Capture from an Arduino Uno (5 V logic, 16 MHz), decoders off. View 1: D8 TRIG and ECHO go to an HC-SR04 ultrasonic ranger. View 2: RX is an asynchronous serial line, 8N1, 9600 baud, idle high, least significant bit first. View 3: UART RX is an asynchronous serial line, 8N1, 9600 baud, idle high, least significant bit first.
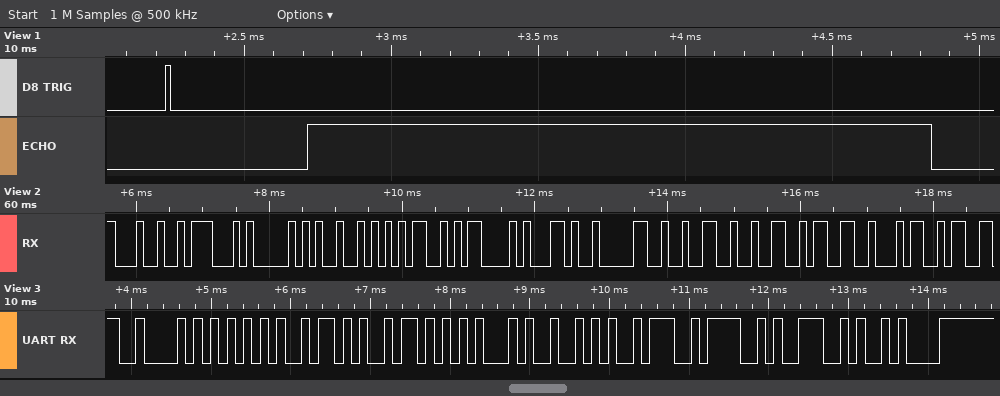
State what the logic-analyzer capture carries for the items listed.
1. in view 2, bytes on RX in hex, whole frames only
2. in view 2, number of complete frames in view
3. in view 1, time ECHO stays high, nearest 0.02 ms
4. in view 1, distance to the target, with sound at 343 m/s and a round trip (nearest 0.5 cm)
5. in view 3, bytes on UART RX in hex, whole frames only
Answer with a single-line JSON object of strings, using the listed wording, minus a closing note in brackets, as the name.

{"in view 2, bytes on RX in hex, whole frames only": "24 47 50 52 4D 43 2C 30 32 32 33 34", "in view 2, number of complete frames in view": "12", "in view 1, time ECHO stays high, nearest 0.02 ms": "2.12 ms", "in view 1, distance to the target, with sound at 343 m/s and a round trip": "36.5 cm", "in view 3, bytes on UART RX in hex, whole frames only": "42 55 5A 5A 45 52 3A 4F 4E 0A"}
